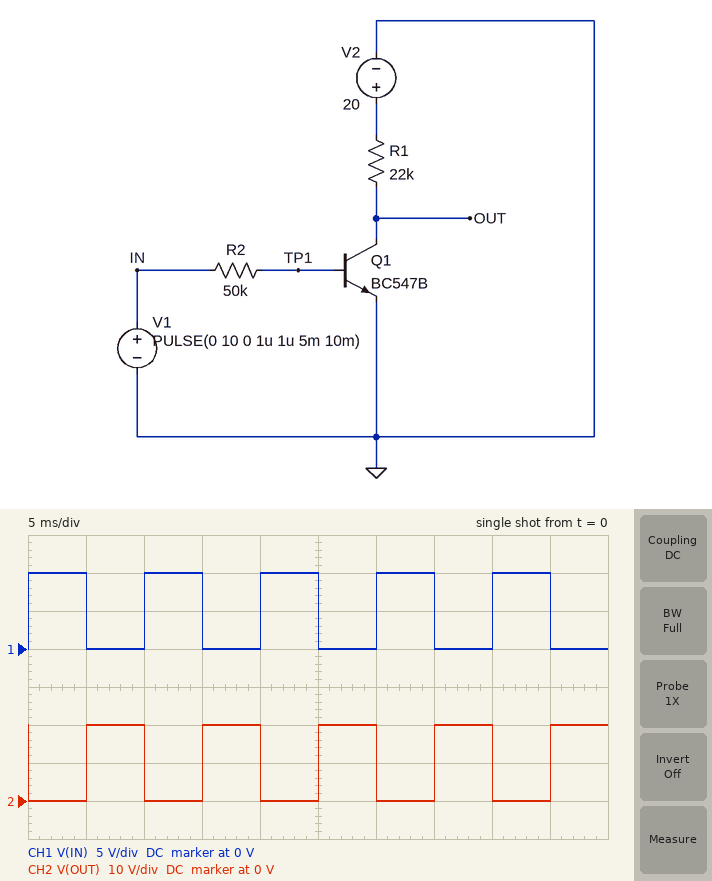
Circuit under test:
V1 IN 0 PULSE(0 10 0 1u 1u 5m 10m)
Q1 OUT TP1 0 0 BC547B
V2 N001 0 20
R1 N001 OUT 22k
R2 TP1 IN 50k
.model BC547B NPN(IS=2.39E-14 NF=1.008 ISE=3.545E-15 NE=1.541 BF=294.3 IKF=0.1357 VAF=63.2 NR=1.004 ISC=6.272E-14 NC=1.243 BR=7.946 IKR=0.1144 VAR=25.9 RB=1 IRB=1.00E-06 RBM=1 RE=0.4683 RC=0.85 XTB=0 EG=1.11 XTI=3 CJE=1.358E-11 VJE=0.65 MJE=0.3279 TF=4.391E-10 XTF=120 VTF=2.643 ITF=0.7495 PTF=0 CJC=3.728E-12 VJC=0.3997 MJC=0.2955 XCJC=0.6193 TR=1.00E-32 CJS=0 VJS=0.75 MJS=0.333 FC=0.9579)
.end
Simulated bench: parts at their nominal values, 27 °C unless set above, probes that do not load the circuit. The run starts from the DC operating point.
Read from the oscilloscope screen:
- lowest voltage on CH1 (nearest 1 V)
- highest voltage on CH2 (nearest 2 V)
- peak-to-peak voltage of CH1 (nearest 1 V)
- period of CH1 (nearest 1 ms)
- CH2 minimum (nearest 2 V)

0 V
20 V
10 V
10 ms
0 V
